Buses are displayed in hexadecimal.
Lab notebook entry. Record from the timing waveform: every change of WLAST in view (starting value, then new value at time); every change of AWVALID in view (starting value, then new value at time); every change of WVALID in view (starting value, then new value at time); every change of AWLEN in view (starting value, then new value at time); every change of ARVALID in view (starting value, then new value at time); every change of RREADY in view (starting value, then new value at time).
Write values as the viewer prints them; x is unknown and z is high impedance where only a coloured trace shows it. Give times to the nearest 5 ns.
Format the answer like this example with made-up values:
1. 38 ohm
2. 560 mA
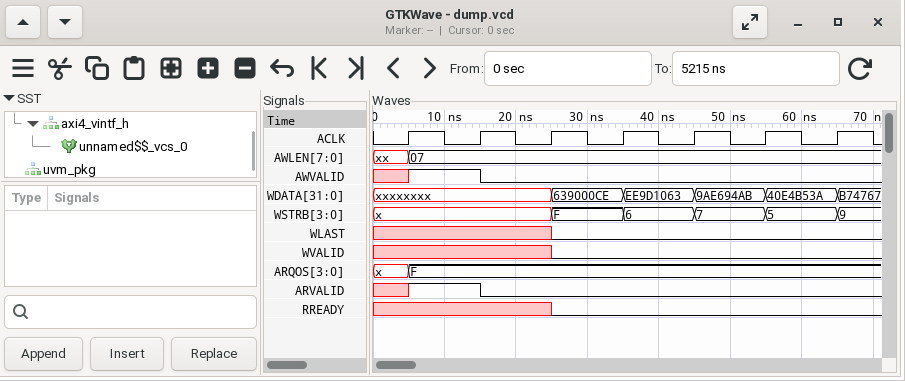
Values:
1. x, 0 at 25 ns
2. x, 1 at 5 ns, 0 at 15 ns
3. x, 0 at 25 ns
4. xx, 07 at 5 ns
5. x, 1 at 5 ns, 0 at 15 ns
6. x, 0 at 25 ns
